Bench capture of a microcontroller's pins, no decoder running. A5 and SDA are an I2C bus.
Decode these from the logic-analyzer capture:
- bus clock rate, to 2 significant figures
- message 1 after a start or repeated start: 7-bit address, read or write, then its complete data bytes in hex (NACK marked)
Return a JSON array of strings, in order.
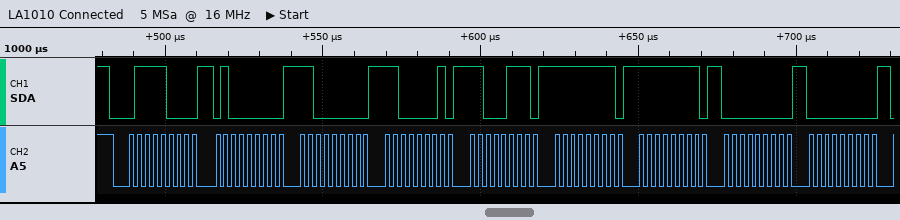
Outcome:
["400 kHz", "0x3C write: 40 C0 C1 C7 FF FF 00 00"]
